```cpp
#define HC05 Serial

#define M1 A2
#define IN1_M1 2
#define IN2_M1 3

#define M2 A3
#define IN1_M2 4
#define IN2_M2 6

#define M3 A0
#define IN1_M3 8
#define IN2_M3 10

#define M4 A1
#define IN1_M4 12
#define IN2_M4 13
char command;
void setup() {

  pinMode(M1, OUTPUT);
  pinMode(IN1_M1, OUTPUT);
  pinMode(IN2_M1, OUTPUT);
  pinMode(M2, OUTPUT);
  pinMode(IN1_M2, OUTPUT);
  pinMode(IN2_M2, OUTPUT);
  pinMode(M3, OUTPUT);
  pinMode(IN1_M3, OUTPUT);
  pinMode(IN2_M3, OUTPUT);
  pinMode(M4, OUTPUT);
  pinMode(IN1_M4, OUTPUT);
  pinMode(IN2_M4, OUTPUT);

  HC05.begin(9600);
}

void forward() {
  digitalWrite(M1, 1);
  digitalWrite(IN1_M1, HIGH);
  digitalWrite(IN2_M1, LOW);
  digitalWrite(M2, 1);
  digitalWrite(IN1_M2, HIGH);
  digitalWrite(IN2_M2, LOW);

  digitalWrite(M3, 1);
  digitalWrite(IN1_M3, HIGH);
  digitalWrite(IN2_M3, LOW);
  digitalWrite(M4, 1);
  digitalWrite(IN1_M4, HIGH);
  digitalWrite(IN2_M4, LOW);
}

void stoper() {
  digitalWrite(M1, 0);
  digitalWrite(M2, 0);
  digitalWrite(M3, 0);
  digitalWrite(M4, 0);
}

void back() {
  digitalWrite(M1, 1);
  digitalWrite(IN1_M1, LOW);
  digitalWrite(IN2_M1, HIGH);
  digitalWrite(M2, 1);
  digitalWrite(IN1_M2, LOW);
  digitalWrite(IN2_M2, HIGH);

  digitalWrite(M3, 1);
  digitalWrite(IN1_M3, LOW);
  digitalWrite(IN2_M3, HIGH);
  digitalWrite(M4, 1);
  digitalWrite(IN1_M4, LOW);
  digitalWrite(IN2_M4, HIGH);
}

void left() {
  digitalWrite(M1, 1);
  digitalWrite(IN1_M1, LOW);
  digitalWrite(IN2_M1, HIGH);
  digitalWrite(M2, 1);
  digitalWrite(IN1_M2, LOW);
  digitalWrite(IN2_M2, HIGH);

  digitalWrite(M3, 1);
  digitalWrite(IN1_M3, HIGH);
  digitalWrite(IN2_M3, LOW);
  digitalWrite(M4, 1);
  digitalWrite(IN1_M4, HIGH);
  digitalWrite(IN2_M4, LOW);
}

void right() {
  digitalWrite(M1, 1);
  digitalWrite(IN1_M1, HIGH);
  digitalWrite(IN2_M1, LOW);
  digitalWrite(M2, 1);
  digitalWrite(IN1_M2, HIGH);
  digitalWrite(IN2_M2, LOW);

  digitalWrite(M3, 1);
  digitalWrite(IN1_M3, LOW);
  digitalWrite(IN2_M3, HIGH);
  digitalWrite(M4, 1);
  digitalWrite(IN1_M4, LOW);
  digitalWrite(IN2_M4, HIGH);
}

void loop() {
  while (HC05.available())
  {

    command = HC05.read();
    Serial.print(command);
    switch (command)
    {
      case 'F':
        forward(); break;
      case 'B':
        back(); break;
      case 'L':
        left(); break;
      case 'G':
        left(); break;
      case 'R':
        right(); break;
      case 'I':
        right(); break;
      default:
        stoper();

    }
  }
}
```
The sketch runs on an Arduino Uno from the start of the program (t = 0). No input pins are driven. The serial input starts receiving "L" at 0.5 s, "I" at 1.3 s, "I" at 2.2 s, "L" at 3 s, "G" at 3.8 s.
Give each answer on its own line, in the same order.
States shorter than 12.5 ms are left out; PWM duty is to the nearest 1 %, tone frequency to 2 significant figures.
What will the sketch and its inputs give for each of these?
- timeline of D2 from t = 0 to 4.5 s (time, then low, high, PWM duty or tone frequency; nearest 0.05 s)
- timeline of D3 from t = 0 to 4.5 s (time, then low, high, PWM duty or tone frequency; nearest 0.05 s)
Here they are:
0 s low; 1.3 s high; 3 s low
0 s low; 0.5 s high; 1.3 s low; 3 s high
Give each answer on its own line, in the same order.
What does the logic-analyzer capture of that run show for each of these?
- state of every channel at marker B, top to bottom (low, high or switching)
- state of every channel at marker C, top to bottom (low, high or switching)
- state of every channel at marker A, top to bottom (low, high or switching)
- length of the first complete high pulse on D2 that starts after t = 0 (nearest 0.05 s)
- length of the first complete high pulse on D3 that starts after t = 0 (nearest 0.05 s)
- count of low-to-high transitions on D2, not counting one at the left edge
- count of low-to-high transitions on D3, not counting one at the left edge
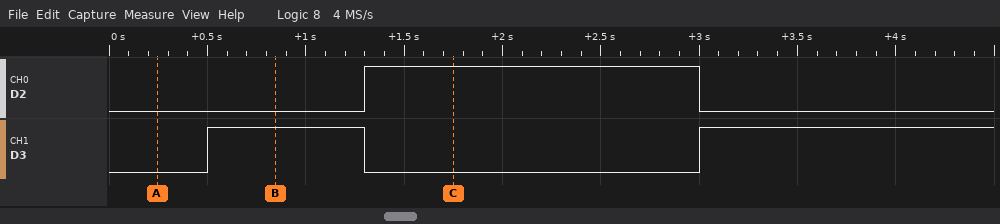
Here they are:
D2 low, D3 high
D2 high, D3 low
D2 low, D3 low
1.70 s
0.80 s
1
2
